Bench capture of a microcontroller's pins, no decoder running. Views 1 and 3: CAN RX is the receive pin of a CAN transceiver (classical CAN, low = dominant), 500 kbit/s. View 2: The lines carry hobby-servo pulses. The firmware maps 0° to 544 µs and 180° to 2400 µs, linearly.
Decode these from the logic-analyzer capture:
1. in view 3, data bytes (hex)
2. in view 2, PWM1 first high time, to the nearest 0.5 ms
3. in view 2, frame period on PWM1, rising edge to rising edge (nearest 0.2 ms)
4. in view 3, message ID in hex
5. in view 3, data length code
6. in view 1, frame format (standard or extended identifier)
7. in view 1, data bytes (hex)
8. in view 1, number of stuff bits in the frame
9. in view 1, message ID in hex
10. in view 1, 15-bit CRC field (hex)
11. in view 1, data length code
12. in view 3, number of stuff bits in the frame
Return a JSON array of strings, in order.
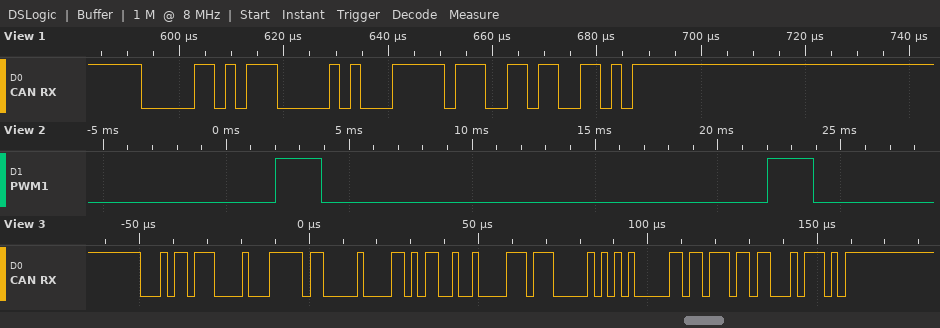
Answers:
["FE 00 D6 48 77 02 A0 B7", "2.0 ms", "20.0 ms", "0x16E", "8", "standard", "1F", "3", "0x057", "0x7366", "1", "4"]
